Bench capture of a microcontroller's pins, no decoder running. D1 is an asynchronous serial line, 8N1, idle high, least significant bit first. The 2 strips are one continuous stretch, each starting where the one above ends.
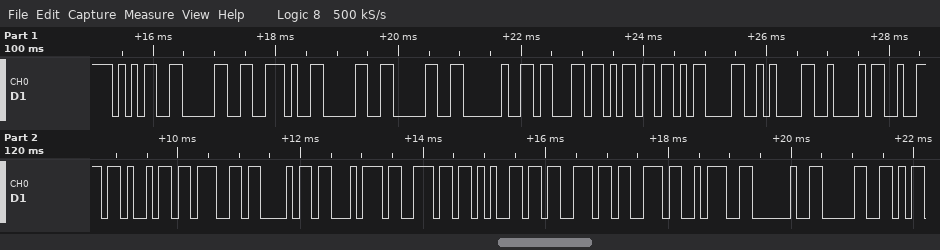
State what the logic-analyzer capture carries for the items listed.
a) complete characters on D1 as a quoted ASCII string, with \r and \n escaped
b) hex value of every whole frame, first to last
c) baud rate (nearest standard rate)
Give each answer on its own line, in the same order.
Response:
"50.00 cm\r\nBrightness: 0"
35 30 2E 30 30 20 63 6D 0D 0A 42 72 69 67 68 74 6E 65 73 73 3A 20 30
9600 baud
